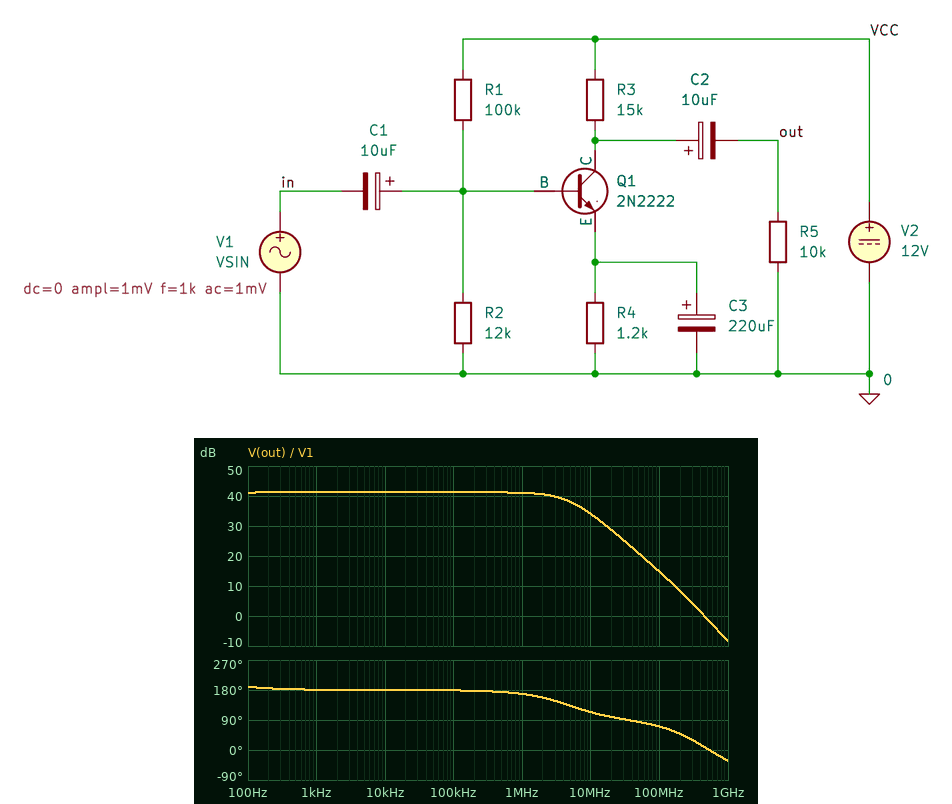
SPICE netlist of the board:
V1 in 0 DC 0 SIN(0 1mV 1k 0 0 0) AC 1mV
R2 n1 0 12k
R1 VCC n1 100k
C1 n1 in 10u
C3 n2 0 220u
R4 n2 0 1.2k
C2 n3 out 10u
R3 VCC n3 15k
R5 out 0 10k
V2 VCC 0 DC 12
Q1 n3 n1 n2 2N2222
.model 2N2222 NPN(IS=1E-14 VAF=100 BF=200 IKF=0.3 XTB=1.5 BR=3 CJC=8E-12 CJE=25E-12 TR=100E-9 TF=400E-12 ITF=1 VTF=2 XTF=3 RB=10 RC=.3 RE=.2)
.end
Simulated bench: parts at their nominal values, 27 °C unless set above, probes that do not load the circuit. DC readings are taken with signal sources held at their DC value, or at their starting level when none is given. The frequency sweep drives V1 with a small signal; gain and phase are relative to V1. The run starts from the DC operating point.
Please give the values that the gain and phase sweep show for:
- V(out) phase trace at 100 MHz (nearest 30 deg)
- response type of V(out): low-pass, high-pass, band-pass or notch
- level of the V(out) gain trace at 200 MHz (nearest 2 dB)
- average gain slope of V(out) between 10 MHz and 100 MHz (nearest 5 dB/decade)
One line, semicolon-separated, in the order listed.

60 deg; low-pass; 8 dB; -20 dB/decade
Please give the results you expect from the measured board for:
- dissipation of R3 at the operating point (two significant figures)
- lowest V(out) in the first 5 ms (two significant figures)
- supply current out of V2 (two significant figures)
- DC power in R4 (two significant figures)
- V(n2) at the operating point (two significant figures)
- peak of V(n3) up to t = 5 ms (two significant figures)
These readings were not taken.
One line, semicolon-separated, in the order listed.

4.0 mW; -120 mV; 620 µA; 320 µW; 620 mV; 4.4 V
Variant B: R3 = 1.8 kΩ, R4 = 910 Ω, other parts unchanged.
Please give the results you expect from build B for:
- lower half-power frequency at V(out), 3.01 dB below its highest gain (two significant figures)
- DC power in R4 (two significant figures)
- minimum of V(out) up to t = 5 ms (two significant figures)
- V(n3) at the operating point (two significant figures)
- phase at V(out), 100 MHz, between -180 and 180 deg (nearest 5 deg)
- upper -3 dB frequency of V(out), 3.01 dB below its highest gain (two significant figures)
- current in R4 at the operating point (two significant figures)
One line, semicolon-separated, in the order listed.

21 Hz; 410 µW; -39 mV; 11 V; 85 deg; 24 MHz; 670 µA
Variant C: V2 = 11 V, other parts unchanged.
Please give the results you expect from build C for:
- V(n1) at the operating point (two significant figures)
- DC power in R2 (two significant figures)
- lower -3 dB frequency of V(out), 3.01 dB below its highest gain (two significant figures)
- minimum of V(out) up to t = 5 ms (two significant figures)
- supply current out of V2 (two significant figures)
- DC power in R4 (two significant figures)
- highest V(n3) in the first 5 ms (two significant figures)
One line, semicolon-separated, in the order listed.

1.2 V; 110 µW; 14 Hz; -98 mV; 530 µA; 230 µW; 4.6 V
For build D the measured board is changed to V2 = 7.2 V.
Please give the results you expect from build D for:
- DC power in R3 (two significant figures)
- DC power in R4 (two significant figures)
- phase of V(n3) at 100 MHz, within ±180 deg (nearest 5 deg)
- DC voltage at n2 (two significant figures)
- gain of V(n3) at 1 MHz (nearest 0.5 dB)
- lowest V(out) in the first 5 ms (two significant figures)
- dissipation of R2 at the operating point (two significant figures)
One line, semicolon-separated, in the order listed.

270 µW; 22 µW; 55 deg; 160 mV; 29.5 dB; -31 mV; 49 µW
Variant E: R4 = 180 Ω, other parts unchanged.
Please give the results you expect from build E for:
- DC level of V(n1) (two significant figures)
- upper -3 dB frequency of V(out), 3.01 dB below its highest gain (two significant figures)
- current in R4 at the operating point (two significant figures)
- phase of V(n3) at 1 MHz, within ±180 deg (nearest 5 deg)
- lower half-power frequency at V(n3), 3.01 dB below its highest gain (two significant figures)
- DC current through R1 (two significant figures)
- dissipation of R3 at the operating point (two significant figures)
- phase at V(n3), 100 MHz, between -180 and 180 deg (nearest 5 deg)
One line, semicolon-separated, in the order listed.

800 mV; 1.7 MHz; 830 µA; 145 deg; 140 Hz; 110 µA; 9.3 mW; -5 deg
